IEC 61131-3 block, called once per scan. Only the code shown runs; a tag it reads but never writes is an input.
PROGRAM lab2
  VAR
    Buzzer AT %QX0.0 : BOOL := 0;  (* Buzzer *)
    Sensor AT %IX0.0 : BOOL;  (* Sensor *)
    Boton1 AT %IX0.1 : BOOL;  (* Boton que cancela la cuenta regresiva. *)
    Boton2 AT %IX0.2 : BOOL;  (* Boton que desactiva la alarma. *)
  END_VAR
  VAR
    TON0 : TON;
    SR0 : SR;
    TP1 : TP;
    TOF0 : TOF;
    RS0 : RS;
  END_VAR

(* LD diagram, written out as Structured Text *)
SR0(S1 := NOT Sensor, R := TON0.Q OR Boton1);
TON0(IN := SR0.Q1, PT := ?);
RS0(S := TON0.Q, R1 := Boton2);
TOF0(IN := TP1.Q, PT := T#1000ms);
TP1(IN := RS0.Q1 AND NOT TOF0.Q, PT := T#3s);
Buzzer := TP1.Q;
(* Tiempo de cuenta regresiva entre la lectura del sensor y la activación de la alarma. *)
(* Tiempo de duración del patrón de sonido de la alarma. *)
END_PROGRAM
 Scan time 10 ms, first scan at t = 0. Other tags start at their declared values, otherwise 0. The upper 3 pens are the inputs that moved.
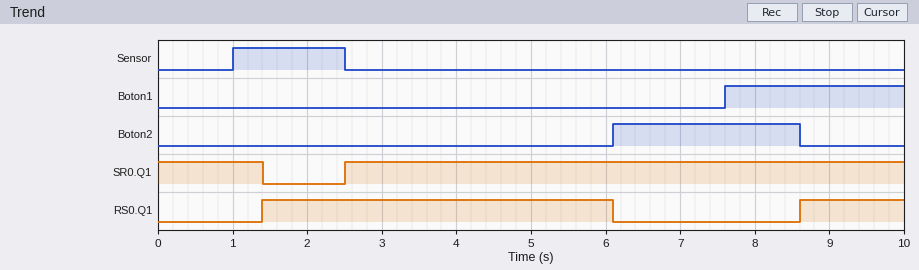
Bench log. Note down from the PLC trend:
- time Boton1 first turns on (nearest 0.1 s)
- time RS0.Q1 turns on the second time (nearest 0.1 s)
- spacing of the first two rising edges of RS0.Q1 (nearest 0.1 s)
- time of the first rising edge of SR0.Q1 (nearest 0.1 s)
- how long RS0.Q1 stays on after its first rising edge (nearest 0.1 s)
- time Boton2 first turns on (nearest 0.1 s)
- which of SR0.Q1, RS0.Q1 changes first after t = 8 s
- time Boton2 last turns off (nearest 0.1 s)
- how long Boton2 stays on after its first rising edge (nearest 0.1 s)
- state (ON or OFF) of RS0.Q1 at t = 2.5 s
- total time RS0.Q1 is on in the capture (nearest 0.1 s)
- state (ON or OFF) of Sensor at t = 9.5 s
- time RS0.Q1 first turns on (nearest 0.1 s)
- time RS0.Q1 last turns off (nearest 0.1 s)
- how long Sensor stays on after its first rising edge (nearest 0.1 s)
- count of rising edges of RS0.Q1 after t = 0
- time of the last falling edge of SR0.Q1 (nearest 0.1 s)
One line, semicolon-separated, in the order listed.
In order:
7.6 s; 8.6 s; 7.2 s; 2.5 s; 4.7 s; 6.1 s; RS0.Q1; 8.6 s; 2.5 s; ON; 6.1 s; OFF; 1.4 s; 6.1 s; 1.5 s; 2; 1.4 s
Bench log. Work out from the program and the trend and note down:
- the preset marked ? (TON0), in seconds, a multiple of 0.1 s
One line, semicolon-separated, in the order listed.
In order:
1.4 s
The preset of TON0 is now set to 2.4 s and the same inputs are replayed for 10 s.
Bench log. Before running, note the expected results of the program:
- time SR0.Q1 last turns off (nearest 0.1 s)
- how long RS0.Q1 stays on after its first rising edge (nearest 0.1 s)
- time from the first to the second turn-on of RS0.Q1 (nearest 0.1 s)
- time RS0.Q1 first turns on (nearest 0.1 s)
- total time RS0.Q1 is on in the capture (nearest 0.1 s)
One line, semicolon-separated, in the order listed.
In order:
2.4 s; 3.7 s; 6.2 s; 2.4 s; 5.1 s
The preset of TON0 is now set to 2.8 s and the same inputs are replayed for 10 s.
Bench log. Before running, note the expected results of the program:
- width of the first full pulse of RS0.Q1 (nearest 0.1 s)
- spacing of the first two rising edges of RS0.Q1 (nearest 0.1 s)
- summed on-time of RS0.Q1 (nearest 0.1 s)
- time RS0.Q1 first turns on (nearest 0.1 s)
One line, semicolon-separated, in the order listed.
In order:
3.3 s; 5.8 s; 4.7 s; 2.8 s
